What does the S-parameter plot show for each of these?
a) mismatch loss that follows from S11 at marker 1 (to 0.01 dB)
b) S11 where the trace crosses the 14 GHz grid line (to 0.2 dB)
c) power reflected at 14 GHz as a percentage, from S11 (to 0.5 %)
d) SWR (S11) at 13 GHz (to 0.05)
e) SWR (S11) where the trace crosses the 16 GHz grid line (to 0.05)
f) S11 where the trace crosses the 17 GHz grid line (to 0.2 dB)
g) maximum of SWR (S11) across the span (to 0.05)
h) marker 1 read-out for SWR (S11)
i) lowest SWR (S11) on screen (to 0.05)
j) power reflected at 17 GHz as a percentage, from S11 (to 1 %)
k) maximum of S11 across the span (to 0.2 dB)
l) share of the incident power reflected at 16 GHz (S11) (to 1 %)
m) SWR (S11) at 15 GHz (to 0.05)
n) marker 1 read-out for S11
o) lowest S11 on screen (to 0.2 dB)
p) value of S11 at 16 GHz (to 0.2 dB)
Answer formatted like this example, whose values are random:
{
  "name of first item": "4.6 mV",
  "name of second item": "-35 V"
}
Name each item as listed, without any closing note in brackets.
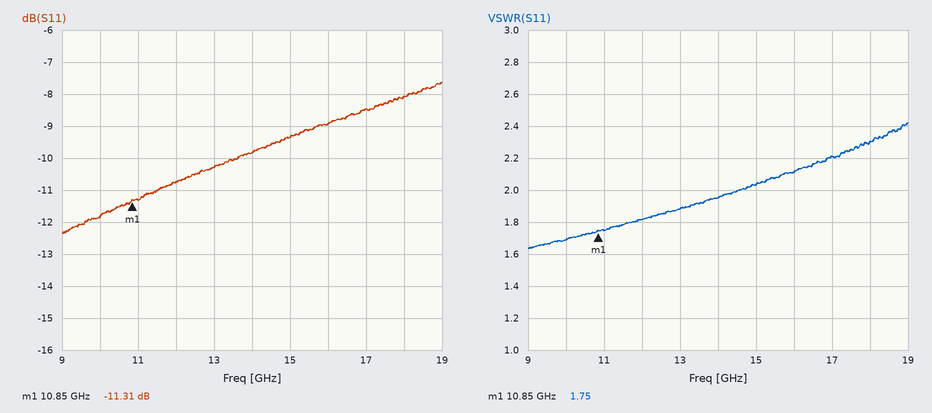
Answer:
{
  "mismatch loss that follows from S11 at marker 1": "0.33 dB",
  "S11 where the trace crosses the 14 GHz grid line": "-9.8 dB",
  "power reflected at 14 GHz as a percentage, from S11": "10.5 %",
  "SWR (S11) at 13 GHz": "1.90",
  "SWR (S11) where the trace crosses the 16 GHz grid line": "2.10",
  "S11 where the trace crosses the 17 GHz grid line": "-8.4 dB",
  "maximum of SWR (S11) across the span": "2.40",
  "marker 1 read-out for SWR": "1.75",
  "lowest SWR (S11) on screen": "1.65",
  "power reflected at 17 GHz as a percentage, from S11": "14 %",
  "maximum of S11 across the span": "-7.6 dB",
  "share of the incident power reflected at 16 GHz (S11)": "13 %",
  "SWR (S11) at 15 GHz": "2.05",
  "marker 1 read-out for S11": "-11.31 dB",
  "lowest S11 on screen": "-12.4 dB",
  "value of S11 at 16 GHz": "-9.0 dB"
}
